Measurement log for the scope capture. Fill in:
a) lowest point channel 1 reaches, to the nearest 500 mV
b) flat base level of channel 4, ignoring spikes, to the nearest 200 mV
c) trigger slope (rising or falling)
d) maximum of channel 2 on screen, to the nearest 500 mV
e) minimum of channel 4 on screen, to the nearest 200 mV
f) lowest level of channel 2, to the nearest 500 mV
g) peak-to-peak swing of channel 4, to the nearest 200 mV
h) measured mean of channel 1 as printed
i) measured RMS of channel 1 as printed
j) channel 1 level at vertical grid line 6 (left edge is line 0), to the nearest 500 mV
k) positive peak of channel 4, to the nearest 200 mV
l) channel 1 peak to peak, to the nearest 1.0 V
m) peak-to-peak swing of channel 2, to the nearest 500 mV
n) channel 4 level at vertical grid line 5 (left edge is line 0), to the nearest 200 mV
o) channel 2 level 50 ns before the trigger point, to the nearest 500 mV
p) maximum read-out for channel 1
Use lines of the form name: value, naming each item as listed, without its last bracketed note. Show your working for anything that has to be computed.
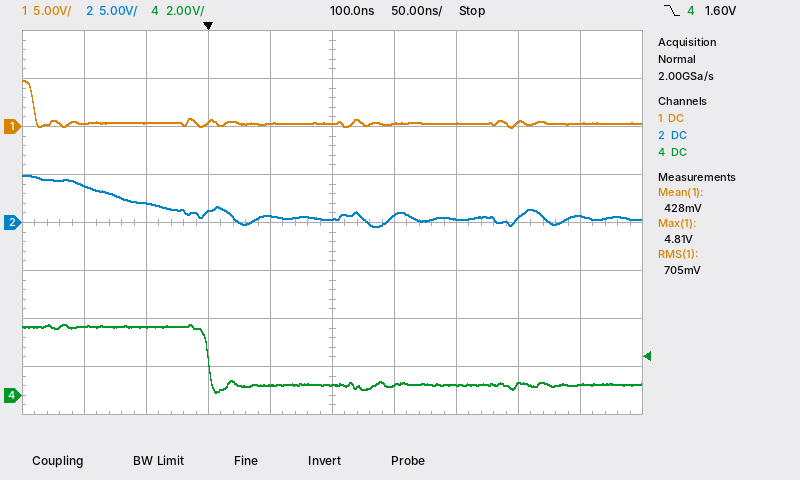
lowest point channel 1 reaches, to the nearest 500 mV: 0.0 V
flat base level of channel 4, ignoring spikes, to the nearest 200 mV: 400 mV
trigger slope: falling
maximum of channel 2 on screen, to the nearest 500 mV: 5.0 V
minimum of channel 4 on screen, to the nearest 200 mV: 200 mV
lowest level of channel 2, to the nearest 500 mV: -500 mV
peak-to-peak swing of channel 4, to the nearest 200 mV: 3.0 V − (200 mV) = 2.8 V
measured mean of channel 1 as printed: 428 mV
measured RMS of channel 1 as printed: 705 mV
channel 1 level at vertical grid line 6 (left edge is line 0), to the nearest 500 mV: 500 mV
positive peak of channel 4, to the nearest 200 mV: 3.0 V
channel 1 peak to peak, to the nearest 1.0 V: 5.0 V
peak-to-peak swing of channel 2, to the nearest 500 mV: 5.0 V − (-500 mV) = 5.5 V
channel 4 level at vertical grid line 5 (left edge is line 0), to the nearest 200 mV: 400 mV
channel 2 level 50 ns before the trigger point, to the nearest 500 mV: 2.0 V
maximum read-out for channel 1: 4.81 V
